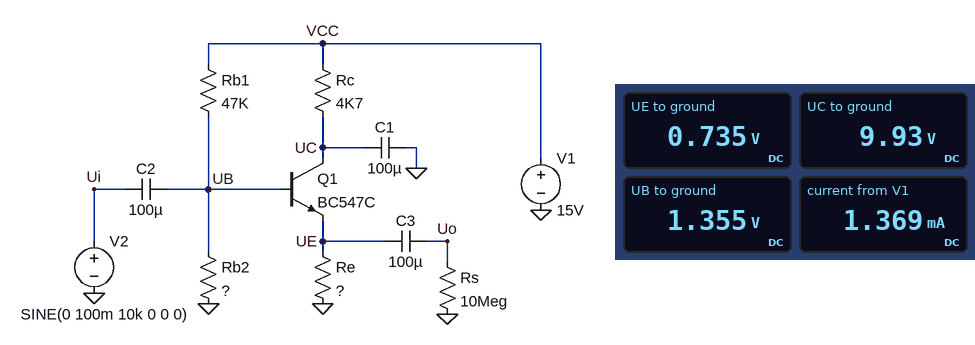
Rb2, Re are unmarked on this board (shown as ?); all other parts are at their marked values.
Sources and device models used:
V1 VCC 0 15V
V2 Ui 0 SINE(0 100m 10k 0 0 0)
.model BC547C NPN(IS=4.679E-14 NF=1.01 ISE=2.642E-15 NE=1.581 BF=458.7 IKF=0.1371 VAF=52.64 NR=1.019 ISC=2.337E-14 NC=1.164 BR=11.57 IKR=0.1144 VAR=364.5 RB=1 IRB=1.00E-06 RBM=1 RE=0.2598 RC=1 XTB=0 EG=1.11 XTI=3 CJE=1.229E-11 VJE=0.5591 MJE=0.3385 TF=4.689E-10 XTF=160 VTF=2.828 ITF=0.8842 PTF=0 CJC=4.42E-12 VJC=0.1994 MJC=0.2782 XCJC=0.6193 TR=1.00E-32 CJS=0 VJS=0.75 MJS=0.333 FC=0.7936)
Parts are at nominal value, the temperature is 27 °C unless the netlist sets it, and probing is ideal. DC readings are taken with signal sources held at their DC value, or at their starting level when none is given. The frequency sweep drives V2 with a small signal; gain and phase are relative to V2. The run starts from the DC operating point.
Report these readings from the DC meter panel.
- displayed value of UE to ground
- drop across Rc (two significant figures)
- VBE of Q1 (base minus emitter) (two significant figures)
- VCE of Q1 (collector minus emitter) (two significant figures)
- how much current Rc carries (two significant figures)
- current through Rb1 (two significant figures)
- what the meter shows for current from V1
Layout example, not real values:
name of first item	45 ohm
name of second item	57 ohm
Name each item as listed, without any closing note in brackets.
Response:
displayed value of UE to ground	0.735 V
drop across Rc	5.1 V
VBE of Q1 (base minus emitter)	620 mV
VCE of Q1 (collector minus emitter)	9.2 V
how much current Rc carries	1.1 mA
current through Rb1	290 µA
what the meter shows for current from V1	1.369 mA
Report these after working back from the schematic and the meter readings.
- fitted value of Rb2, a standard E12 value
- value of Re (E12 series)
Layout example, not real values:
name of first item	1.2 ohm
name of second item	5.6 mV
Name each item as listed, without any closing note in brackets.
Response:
fitted value of Rb2, a standard E12 value	4.7 kΩ
value of Re	680 Ω
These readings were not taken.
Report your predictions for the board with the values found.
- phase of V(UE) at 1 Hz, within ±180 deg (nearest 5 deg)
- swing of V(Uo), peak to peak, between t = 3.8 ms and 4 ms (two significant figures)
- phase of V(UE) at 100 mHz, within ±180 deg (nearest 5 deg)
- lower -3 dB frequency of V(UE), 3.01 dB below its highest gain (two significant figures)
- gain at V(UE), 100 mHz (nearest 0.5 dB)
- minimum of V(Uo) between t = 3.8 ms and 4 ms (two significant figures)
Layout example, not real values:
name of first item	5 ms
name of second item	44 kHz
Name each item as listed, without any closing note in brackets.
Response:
phase of V(UE) at 1 Hz, within ±180 deg	20 deg
swing of V(Uo), peak to peak, between t = 3.8 ms and 4 ms	190 mV
phase of V(UE) at 100 mHz, within ±180 deg	75 deg
lower -3 dB frequency of V(UE), 3.01 dB below its highest gain	380 mHz
gain at V(UE), 100 mHz	-12.0 dB
minimum of V(Uo) between t = 3.8 ms and 4 ms	-96 mV
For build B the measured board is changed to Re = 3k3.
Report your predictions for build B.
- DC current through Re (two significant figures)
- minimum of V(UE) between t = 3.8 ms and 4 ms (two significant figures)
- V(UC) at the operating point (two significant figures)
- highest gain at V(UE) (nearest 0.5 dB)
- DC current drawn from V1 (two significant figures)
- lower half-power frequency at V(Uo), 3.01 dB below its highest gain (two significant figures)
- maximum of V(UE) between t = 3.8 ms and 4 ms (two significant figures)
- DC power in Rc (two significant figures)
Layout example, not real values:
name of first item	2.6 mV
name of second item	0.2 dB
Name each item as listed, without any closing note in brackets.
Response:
DC current through Re	240 µA
minimum of V(UE) between t = 3.8 ms and 4 ms	690 mV
V(UC) at the operating point	14 V
highest gain at V(UE)	-0.5 dB
DC current drawn from V1	530 µA
lower half-power frequency at V(Uo), 3.01 dB below its highest gain	370 mHz
maximum of V(UE) between t = 3.8 ms and 4 ms	880 mV
DC power in Rc	260 µW
